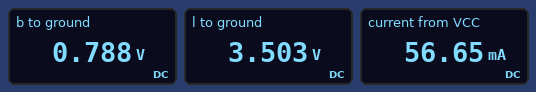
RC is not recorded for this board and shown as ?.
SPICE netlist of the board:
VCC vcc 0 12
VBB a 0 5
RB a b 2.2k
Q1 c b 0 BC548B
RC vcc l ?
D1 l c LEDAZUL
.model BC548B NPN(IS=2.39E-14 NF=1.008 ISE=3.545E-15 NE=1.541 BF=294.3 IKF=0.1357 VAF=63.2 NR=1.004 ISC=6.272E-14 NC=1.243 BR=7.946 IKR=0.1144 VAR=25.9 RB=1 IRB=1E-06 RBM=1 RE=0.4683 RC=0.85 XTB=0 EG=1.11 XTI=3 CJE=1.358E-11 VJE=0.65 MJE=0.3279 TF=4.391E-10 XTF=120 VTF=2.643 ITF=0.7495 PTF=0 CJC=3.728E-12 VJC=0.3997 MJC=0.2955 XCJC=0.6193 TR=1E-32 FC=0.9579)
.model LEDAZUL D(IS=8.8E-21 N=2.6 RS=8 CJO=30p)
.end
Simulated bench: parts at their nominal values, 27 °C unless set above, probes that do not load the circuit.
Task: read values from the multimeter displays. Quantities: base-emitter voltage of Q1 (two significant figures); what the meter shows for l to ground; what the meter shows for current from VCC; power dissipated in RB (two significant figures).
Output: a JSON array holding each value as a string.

["790 mV", "3.503 V", "56.65 mA", "8.1 mW"]
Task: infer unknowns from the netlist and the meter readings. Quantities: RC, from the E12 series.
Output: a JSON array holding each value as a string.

["150 Ω"]
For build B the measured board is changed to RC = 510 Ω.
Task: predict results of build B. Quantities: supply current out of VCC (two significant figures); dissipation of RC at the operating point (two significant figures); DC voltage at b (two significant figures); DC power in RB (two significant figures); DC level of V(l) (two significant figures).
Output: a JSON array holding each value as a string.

["18 mA", "160 mW", "740 mV", "8.2 mW", "3.0 V"]
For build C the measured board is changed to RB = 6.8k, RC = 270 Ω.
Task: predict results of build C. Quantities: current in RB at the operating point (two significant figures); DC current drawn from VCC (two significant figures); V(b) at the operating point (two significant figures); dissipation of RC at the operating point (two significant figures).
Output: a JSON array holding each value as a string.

["620 µA", "32 mA", "750 mV", "280 mW"]
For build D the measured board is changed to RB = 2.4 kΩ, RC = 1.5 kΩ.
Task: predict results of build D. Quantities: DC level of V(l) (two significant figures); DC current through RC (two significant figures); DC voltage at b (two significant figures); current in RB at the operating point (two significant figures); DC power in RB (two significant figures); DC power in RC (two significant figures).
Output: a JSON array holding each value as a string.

["2.8 V", "6.1 mA", "720 mV", "1.8 mA", "7.6 mW", "56 mW"]
